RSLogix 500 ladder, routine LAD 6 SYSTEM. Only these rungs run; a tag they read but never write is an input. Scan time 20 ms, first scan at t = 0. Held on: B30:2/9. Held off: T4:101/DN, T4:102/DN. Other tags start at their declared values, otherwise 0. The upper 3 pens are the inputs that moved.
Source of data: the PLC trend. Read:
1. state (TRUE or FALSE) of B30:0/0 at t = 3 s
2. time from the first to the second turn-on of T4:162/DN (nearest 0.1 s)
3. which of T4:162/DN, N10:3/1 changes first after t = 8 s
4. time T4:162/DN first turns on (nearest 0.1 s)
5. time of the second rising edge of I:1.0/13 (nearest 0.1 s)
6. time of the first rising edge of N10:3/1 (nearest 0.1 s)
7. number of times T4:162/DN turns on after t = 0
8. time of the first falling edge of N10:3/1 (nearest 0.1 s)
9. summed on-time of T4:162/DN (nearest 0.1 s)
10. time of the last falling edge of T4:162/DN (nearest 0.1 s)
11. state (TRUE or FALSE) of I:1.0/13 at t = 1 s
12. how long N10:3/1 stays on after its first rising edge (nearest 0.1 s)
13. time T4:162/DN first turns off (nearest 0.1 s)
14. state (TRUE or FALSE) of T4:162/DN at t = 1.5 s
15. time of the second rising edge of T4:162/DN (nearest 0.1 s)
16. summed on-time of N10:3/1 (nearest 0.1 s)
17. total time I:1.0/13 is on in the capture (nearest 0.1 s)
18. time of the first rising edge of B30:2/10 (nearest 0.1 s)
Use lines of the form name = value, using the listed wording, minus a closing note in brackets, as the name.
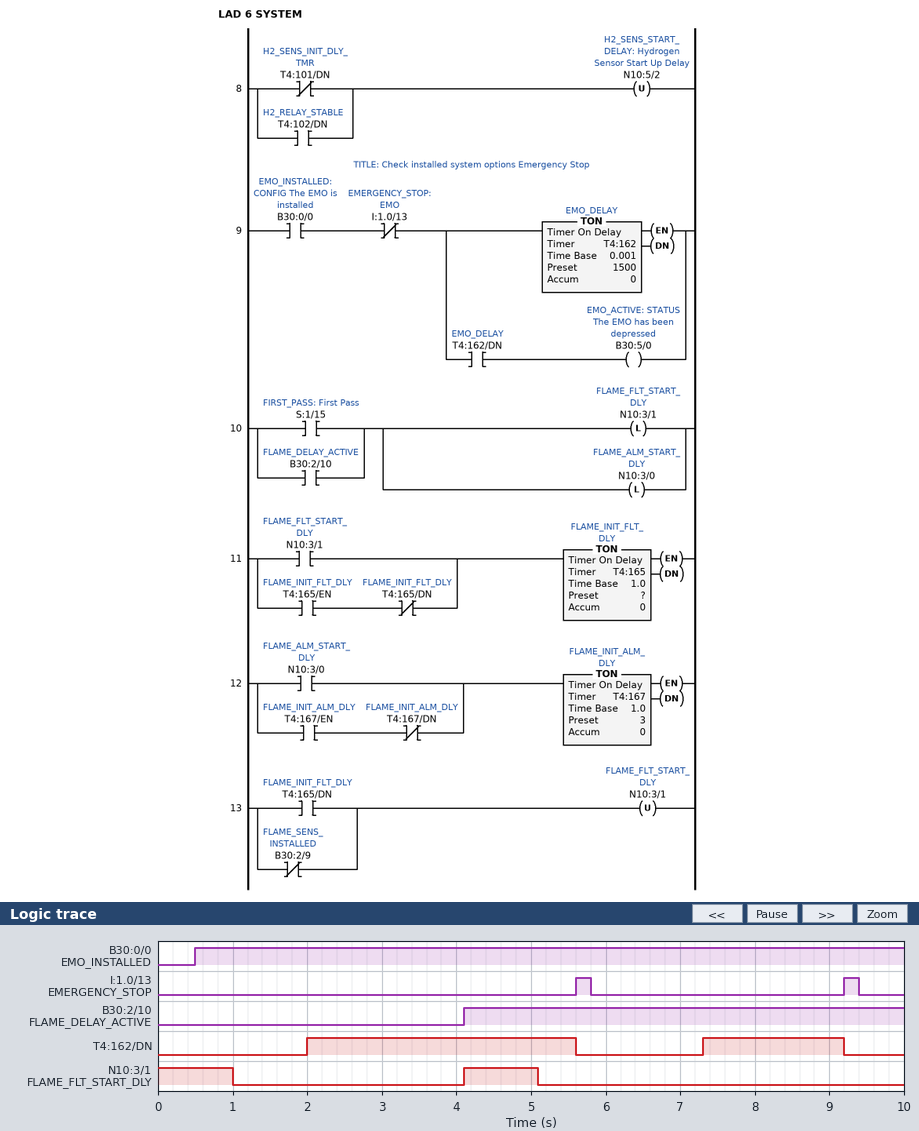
state (TRUE or FALSE) of B30:0/0 at t = 3 s = TRUE
time from the first to the second turn-on of T4:162/DN = 5.3 s
which of T4:162/DN, N10:3/1 changes first after t = 8 s = T4:162/DN
time T4:162/DN first turns on = 2.0 s
time of the second rising edge of I:1.0/13 = 9.2 s
time of the first rising edge of N10:3/1 = 4.1 s
number of times T4:162/DN turns on after t = 0 = 2
time of the first falling edge of N10:3/1 = 1.0 s
summed on-time of T4:162/DN = 5.5 s
time of the last falling edge of T4:162/DN = 9.2 s
state (TRUE or FALSE) of I:1.0/13 at t = 1 s = FALSE
how long N10:3/1 stays on after its first rising edge = 1.0 s
time T4:162/DN first turns off = 5.6 s
state (TRUE or FALSE) of T4:162/DN at t = 1.5 s = FALSE
time of the second rising edge of T4:162/DN = 7.3 s
summed on-time of N10:3/1 = 2.0 s
total time I:1.0/13 is on in the capture = 0.4 s
time of the first rising edge of B30:2/10 = 4.1 s
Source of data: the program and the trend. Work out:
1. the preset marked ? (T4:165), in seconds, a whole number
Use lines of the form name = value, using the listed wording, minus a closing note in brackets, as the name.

the preset marked ? (T4:165), in seconds, a whole number = 1 s
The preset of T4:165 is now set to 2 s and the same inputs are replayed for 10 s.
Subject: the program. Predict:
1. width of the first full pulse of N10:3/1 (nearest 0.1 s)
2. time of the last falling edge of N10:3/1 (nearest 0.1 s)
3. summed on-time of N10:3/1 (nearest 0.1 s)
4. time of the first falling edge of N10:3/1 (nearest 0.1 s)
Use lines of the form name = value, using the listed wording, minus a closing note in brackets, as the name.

width of the first full pulse of N10:3/1 = 2.0 s
time of the last falling edge of N10:3/1 = 6.1 s
summed on-time of N10:3/1 = 4.0 s
time of the first falling edge of N10:3/1 = 2.0 s
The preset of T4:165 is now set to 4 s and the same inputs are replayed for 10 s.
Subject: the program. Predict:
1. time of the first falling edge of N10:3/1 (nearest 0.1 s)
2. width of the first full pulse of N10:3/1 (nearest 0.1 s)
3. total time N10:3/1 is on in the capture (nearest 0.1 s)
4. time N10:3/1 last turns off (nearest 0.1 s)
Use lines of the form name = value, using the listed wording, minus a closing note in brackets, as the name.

time of the first falling edge of N10:3/1 = 4.0 s
width of the first full pulse of N10:3/1 = 4.0 s
total time N10:3/1 is on in the capture = 8.0 s
time N10:3/1 last turns off = 8.1 s
